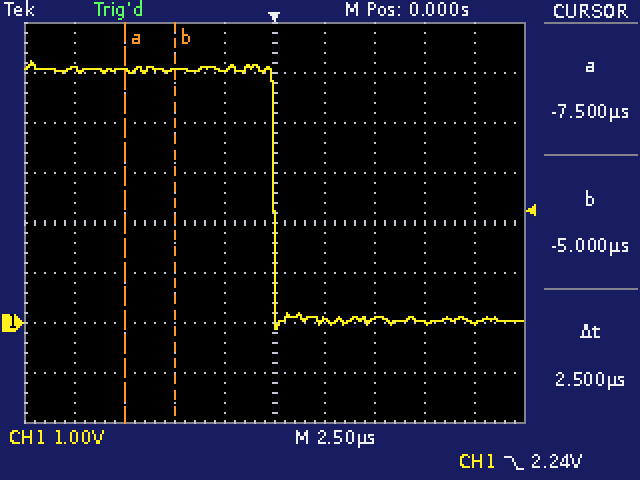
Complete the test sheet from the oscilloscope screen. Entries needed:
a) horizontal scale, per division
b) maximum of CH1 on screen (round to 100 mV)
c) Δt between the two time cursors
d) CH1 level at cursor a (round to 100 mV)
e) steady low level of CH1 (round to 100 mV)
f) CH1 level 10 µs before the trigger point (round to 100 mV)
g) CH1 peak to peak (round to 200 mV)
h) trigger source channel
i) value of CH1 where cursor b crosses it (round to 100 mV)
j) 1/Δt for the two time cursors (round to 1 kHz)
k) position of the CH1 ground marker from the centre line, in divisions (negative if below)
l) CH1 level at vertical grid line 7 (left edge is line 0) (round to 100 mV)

2.5 µs
5.2 V
2.5 µs
5.0 V
100 mV
5.1 V
5.4 V
CH1
5.1 V
400 kHz
-2.0 div
100 mV
